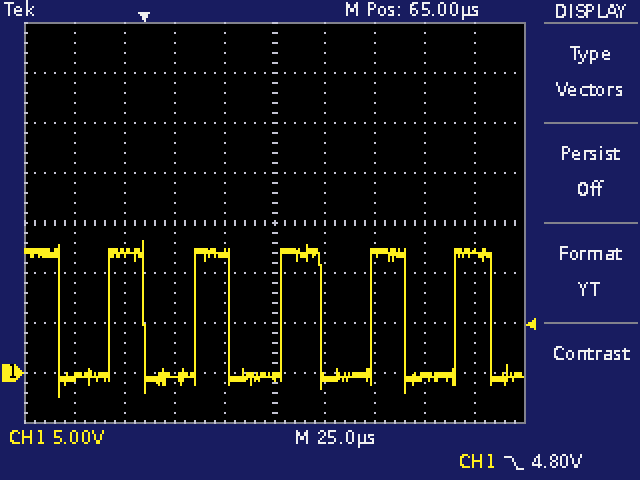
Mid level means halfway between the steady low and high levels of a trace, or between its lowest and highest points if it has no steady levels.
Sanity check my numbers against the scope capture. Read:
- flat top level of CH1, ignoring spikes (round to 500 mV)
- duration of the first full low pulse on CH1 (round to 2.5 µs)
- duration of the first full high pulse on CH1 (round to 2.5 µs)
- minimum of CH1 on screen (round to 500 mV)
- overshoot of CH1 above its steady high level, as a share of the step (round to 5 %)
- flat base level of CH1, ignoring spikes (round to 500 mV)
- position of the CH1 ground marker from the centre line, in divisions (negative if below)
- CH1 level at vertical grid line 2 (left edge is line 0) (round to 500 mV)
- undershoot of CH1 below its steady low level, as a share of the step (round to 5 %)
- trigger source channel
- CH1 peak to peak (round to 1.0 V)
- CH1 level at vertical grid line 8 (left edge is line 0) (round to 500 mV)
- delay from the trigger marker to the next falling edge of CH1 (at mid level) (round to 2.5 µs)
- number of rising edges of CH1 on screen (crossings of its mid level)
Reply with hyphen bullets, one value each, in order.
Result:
- 12.0 V
- 25.0 µs
- 17.5 µs
- -2.5 V
- 10 %
- -500 mV
- -3.0 div
- 12.0 V
- 15 %
- CH1
- 16.0 V
- -500 mV
- 42.5 µs
- 5
